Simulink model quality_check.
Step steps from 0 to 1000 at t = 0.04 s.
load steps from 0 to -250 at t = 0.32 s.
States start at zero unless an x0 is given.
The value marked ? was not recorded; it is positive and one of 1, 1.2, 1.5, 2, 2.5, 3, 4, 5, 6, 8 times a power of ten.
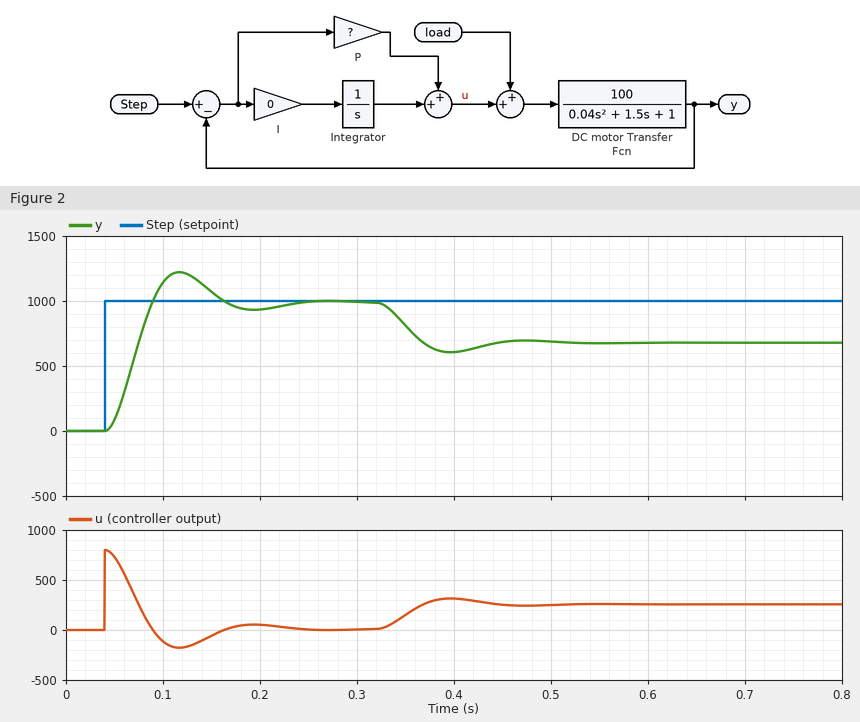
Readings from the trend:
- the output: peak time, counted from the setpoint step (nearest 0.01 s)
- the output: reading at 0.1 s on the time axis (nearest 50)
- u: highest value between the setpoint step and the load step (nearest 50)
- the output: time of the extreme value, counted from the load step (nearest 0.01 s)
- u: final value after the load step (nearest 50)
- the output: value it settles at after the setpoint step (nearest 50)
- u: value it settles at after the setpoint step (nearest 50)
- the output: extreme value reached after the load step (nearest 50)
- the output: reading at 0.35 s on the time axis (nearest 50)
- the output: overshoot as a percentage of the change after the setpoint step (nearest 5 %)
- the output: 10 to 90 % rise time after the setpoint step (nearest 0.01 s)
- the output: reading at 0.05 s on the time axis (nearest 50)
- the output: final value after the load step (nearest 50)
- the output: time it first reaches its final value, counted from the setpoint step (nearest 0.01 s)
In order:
0.08 s
1150
800
0.08 s
250
1000
0
600
800
25 %
0.03 s
100
700
0.05 s
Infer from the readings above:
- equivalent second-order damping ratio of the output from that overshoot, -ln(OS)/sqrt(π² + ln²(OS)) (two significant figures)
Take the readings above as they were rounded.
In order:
0.40
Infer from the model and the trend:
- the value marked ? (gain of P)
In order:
0.8
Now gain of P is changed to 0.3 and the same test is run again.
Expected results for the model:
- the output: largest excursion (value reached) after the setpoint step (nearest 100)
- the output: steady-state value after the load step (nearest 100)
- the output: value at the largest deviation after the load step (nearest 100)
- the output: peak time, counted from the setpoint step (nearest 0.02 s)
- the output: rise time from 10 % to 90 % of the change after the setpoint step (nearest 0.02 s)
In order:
1000
200
100
0.16 s
0.08 s
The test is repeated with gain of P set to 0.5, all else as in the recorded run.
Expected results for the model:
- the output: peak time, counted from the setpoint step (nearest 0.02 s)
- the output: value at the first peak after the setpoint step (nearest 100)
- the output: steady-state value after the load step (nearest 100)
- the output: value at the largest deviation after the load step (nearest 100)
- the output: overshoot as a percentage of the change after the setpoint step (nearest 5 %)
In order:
0.10 s
1100
500
400
15 %
